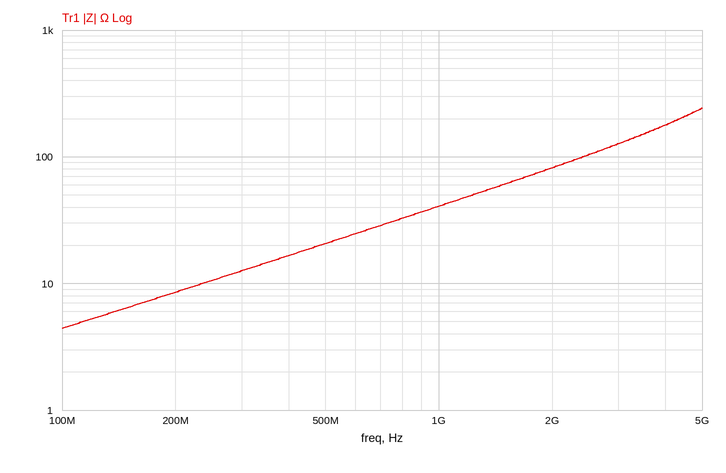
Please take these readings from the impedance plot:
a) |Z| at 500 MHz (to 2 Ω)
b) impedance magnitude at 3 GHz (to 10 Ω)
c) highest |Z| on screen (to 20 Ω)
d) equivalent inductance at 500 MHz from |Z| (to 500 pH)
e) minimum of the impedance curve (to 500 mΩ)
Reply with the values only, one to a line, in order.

20 Ω
130 Ω
240 Ω
6.5 nH
4.5 Ω
